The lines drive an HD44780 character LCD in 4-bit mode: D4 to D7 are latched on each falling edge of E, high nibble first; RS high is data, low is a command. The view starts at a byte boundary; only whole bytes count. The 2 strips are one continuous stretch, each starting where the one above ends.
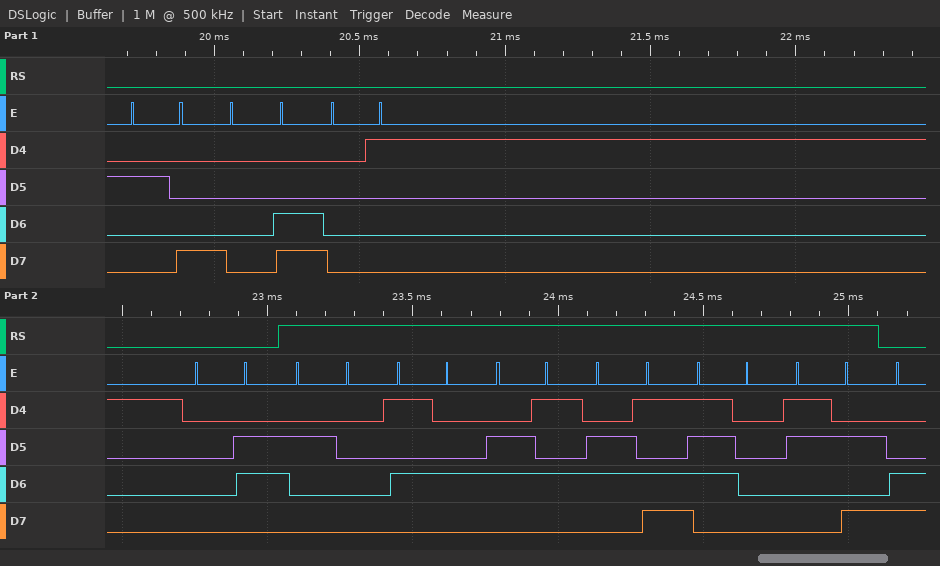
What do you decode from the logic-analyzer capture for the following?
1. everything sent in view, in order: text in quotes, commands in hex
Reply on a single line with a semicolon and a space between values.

0x28 0x0C 0x01 0x06 " Temp:"
